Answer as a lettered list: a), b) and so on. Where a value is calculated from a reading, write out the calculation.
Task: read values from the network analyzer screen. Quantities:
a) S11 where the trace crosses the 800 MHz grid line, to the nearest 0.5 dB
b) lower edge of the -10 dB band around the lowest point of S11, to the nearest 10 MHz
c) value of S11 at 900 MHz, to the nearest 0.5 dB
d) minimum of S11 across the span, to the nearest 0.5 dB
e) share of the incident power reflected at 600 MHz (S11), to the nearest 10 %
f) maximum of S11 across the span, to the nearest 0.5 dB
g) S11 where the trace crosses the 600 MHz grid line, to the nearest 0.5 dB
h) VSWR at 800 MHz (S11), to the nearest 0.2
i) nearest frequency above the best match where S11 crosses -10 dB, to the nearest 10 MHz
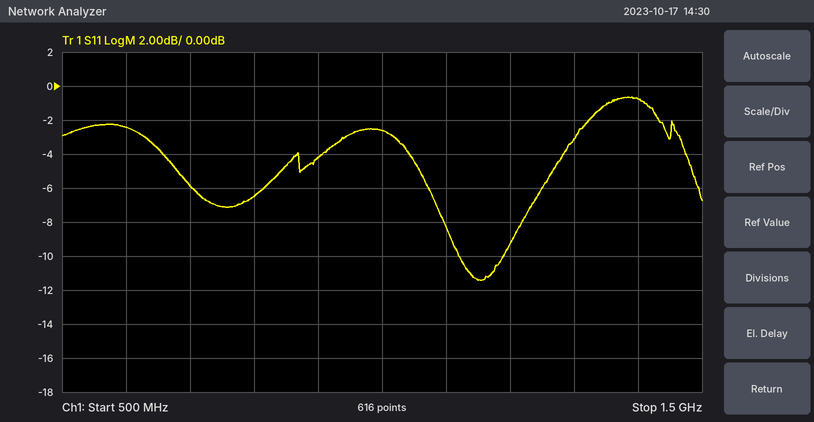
a) -6.5 dB
b) 1.12 GHz
c) -4.0 dB
d) -11.5 dB
e) 10^(-2.5/10) ≈ 56.2 %, so 60 % to the nearest 10 %
f) -0.5 dB
g) -2.5 dB
h) |Γ| = 10^(-6.5/20) = 0.4732; VSWR = (1 + 0.4732)/(1 − 0.4732) ≈ 2.8
i) 1.19 GHz
